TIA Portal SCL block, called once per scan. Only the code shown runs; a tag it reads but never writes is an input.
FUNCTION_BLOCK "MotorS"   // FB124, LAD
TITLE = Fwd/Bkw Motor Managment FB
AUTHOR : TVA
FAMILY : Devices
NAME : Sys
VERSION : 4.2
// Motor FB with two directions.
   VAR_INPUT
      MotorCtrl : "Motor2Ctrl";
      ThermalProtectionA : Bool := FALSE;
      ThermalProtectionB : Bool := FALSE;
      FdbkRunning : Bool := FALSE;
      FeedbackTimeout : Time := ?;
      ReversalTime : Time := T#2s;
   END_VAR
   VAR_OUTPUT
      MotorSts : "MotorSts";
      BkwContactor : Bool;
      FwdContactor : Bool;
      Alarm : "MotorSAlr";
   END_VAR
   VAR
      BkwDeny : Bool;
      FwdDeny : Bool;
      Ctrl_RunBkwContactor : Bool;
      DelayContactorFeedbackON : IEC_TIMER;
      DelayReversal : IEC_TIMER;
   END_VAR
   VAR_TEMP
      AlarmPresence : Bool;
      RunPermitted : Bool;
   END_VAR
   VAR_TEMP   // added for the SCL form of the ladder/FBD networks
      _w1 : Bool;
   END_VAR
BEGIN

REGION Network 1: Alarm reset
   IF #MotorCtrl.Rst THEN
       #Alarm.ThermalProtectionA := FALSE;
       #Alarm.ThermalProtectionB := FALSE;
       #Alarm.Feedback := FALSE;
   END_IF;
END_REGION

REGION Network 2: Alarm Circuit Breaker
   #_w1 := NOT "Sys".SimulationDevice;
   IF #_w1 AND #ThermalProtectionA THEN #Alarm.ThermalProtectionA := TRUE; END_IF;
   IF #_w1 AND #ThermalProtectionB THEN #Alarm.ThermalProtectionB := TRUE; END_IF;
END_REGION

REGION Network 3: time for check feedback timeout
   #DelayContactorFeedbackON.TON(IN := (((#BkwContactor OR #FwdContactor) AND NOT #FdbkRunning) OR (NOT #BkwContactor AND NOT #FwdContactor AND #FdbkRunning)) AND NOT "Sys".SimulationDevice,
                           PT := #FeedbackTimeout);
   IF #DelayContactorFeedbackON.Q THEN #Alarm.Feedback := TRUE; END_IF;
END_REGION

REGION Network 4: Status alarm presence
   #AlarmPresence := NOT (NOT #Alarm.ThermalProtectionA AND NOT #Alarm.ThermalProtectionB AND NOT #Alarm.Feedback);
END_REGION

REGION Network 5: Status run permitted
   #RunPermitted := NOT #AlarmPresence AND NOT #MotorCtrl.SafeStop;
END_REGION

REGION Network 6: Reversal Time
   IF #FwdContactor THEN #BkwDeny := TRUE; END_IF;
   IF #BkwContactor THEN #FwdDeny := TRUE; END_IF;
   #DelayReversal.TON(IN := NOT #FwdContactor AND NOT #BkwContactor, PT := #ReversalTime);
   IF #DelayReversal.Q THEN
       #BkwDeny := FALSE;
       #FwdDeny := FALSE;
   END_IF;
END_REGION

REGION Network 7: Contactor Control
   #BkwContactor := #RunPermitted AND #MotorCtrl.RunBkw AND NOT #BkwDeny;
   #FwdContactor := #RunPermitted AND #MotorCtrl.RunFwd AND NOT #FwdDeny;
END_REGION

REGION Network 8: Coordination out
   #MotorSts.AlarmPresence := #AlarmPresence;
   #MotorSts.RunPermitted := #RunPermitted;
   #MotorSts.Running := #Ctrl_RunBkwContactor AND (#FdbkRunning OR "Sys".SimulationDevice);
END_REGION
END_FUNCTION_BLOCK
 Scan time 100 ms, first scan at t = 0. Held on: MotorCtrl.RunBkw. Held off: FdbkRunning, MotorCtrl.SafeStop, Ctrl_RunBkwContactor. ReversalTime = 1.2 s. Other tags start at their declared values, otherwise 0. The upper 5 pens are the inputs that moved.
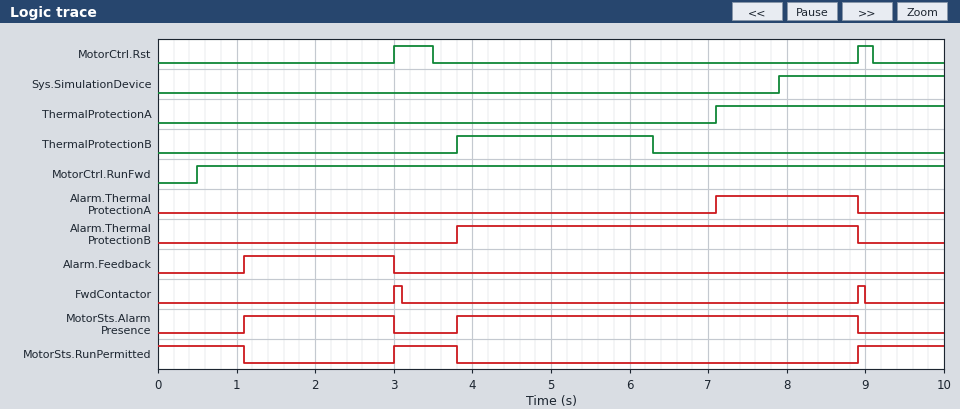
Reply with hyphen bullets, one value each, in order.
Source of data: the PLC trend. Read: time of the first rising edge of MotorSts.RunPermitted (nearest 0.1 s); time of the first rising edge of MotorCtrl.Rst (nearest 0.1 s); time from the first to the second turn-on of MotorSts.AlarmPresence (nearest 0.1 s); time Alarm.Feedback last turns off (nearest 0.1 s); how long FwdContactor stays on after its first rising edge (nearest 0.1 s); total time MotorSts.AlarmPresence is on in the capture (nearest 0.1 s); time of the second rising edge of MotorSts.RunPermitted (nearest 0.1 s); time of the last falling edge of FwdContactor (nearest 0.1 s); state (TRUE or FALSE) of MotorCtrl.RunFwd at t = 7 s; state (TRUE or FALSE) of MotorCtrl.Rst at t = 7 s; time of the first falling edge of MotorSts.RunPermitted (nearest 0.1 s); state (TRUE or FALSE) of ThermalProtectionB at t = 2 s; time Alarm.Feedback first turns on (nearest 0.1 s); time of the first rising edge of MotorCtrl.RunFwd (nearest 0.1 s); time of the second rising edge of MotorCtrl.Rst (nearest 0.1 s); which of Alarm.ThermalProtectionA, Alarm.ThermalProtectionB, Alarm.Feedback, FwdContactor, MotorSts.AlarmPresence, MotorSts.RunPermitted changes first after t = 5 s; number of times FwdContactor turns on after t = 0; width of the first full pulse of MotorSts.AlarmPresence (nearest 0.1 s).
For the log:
- 3.0 s
- 3.0 s
- 2.7 s
- 3.0 s
- 0.1 s
- 7.0 s
- 8.9 s
- 9.0 s
- TRUE
- FALSE
- 1.1 s
- FALSE
- 1.1 s
- 0.5 s
- 8.9 s
- Alarm.ThermalProtectionA
- 2
- 1.9 s
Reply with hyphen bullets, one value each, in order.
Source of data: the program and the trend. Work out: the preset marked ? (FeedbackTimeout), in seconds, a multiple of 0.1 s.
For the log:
- 1.0 s
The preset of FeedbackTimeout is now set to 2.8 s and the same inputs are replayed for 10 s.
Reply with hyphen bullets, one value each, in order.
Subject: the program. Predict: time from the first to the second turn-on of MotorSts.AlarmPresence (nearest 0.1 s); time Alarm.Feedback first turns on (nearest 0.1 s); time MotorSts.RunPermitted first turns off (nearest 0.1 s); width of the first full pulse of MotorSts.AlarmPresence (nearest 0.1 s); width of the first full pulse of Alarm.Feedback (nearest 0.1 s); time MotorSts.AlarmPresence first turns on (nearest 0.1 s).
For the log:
- 0.9 s
- 2.9 s
- 2.9 s
- 0.1 s
- 0.1 s
- 2.9 s
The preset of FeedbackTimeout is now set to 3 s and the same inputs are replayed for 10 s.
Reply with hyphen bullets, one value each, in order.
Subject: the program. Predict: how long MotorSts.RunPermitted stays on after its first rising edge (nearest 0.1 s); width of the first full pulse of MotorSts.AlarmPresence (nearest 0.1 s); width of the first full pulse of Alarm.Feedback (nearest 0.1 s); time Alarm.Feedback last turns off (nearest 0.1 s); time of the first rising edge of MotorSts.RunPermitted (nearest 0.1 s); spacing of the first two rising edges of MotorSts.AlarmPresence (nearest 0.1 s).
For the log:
- 0.6 s
- 0.1 s
- 0.1 s
- 3.2 s
- 3.2 s
- 0.7 s
